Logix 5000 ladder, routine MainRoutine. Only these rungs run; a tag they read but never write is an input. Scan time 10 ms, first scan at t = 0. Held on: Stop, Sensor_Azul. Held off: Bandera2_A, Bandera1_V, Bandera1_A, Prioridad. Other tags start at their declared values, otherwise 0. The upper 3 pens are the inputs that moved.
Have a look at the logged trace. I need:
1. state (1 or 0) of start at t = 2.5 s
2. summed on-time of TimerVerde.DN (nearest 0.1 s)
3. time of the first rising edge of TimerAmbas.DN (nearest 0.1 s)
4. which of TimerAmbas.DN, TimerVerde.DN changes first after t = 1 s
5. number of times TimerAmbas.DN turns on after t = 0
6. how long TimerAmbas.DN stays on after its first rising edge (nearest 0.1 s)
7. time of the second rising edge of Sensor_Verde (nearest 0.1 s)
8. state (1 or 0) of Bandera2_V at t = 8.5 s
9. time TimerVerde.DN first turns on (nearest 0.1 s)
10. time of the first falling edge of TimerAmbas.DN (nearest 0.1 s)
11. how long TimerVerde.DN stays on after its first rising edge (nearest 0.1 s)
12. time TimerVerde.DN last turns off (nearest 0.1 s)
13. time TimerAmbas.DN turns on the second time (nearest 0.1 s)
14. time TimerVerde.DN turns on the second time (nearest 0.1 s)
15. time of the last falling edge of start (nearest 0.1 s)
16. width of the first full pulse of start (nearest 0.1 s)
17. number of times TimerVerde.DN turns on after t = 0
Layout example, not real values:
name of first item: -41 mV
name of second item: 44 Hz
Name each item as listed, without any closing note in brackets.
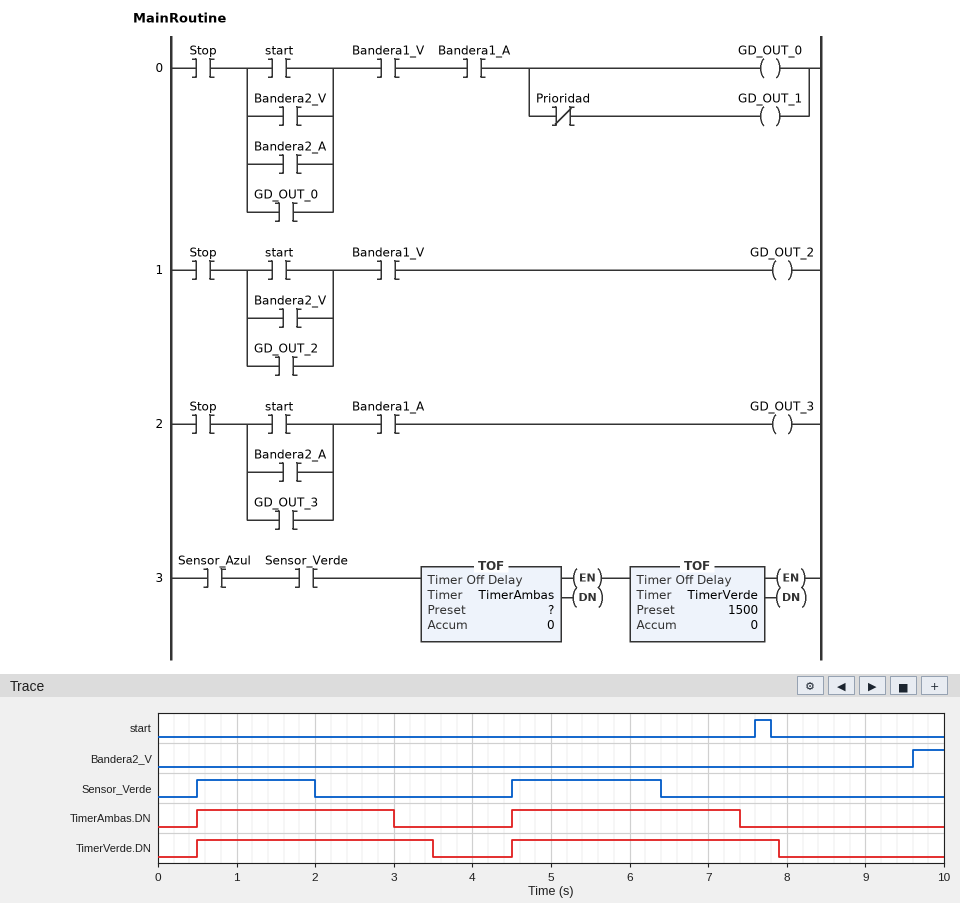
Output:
state (1 or 0) of start at t = 2.5 s: 0
summed on-time of TimerVerde.DN: 6.4 s
time of the first rising edge of TimerAmbas.DN: 0.5 s
which of TimerAmbas.DN, TimerVerde.DN changes first after t = 1 s: TimerAmbas.DN
number of times TimerAmbas.DN turns on after t = 0: 2
how long TimerAmbas.DN stays on after its first rising edge: 2.5 s
time of the second rising edge of Sensor_Verde: 4.5 s
state (1 or 0) of Bandera2_V at t = 8.5 s: 0
time TimerVerde.DN first turns on: 0.5 s
time of the first falling edge of TimerAmbas.DN: 3.0 s
how long TimerVerde.DN stays on after its first rising edge: 3.0 s
time TimerVerde.DN last turns off: 7.9 s
time TimerAmbas.DN turns on the second time: 4.5 s
time TimerVerde.DN turns on the second time: 4.5 s
time of the last falling edge of start: 7.8 s
width of the first full pulse of start: 0.2 s
number of times TimerVerde.DN turns on after t = 0: 2
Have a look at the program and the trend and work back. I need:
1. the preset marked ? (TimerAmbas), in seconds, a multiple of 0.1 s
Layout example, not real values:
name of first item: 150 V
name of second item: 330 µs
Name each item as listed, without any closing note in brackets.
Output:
the preset marked ? (TimerAmbas), in seconds, a multiple of 0.1 s: 1.0 s
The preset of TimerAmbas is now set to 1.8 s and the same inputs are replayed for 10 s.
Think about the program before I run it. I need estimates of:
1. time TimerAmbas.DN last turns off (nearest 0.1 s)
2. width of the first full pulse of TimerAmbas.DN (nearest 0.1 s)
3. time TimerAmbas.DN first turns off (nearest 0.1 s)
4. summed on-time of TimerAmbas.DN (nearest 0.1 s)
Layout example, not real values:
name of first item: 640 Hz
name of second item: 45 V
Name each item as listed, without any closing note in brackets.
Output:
time TimerAmbas.DN last turns off: 8.2 s
width of the first full pulse of TimerAmbas.DN: 3.3 s
time TimerAmbas.DN first turns off: 3.8 s
summed on-time of TimerAmbas.DN: 7.0 s
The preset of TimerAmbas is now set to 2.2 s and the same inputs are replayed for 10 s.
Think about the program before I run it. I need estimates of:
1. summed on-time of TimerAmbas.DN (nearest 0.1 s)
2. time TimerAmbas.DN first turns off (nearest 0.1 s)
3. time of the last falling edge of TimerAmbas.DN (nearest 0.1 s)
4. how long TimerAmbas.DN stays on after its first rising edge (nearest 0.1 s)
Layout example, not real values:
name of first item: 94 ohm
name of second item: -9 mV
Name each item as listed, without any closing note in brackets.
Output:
summed on-time of TimerAmbas.DN: 7.8 s
time TimerAmbas.DN first turns off: 4.2 s
time of the last falling edge of TimerAmbas.DN: 8.6 s
how long TimerAmbas.DN stays on after its first rising edge: 3.7 s
